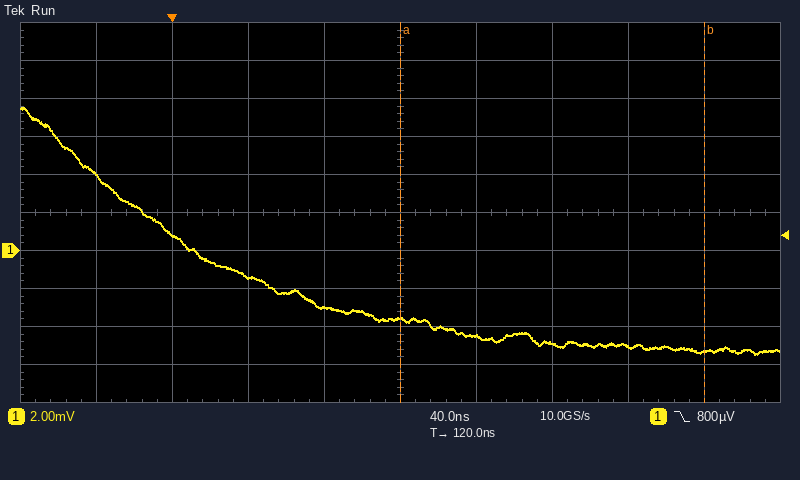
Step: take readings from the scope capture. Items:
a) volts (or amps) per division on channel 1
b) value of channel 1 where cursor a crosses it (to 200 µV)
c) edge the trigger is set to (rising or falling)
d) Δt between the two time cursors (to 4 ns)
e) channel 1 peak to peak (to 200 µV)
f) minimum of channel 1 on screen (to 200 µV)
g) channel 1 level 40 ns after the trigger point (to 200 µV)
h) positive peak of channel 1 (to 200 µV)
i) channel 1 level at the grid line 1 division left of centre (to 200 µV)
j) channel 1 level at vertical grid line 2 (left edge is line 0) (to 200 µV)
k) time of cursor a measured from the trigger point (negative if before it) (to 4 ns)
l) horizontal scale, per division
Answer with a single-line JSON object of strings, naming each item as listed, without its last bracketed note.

{"volts (or amps) per division on channel 1": "2 mV", "value of channel 1 where cursor a crosses it": "-3.6 mV", "edge the trigger is set to": "falling", "Δt between the two time cursors": "160 ns", "channel 1 peak to peak": "13.0 mV", "minimum of channel 1 on screen": "-5.4 mV", "channel 1 level 40 ns after the trigger point": "-1.4 mV", "positive peak of channel 1": "7.6 mV", "channel 1 level at the grid line 1 division left of centre": "-3.0 mV", "channel 1 level at vertical grid line 2 (left edge is line 0)": "800 µV", "time of cursor a measured from the trigger point (negative if before it)": "+120 ns", "horizontal scale, per division": "40 ns"}
